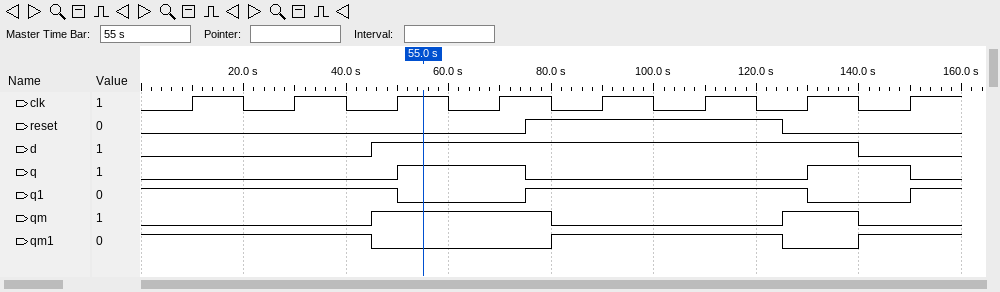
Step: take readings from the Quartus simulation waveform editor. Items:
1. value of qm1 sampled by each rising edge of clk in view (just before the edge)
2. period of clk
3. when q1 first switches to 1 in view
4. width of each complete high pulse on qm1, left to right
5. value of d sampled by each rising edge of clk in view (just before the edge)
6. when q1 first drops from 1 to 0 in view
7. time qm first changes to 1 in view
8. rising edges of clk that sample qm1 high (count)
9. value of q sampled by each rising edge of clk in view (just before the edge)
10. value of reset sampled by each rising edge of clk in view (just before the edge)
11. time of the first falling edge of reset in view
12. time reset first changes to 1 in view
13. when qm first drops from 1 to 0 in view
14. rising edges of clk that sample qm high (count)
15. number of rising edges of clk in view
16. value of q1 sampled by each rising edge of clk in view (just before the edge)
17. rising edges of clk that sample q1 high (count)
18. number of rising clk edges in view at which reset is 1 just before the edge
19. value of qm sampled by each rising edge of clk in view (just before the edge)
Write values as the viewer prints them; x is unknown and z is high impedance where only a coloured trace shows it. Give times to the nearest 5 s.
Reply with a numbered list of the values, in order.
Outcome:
1. 1 1 0 0 1 1 0 1
2. 20 s
3. 75 s
4. 45 s
5. 0 0 1 1 1 1 1 0
6. 50 s
7. 45 s
8. 5
9. 0 0 0 1 0 0 0 1
10. 0 0 0 0 1 1 0 0
11. 125 s
12. 75 s
13. 80 s
14. 3
15. 8
16. 1 1 1 0 1 1 1 0
17. 6
18. 2
19. 0 0 1 1 0 0 1 0
